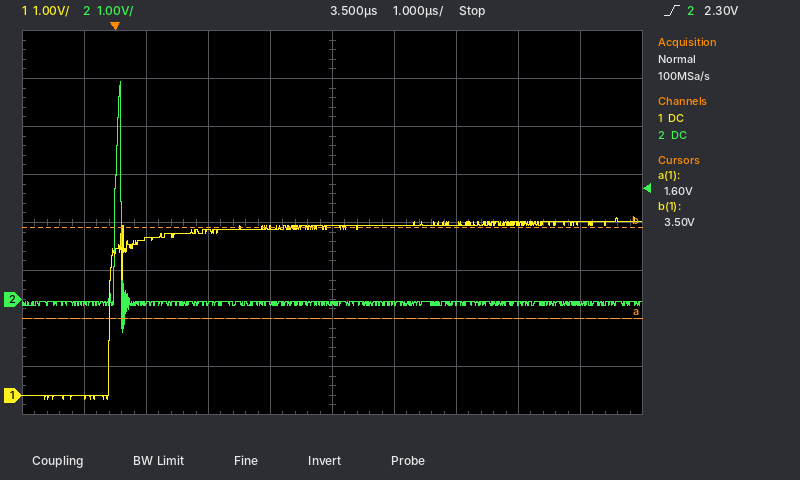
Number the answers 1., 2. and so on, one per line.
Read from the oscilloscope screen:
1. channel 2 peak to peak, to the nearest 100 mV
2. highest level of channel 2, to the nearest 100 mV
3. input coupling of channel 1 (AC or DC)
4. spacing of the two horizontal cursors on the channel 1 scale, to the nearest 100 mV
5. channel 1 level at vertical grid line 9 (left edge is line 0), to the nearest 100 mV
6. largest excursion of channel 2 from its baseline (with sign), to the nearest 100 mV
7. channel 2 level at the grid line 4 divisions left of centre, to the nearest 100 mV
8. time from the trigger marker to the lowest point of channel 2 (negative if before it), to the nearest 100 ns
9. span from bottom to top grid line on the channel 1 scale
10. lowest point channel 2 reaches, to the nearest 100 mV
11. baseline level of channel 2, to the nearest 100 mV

1. 5.2 V
2. 4.5 V
3. DC
4. 1.9 V
5. 3.6 V
6. +4.6 V
7. -100 mV
8. +100 ns
9. 8 V
10. -700 mV
11. -100 mV
